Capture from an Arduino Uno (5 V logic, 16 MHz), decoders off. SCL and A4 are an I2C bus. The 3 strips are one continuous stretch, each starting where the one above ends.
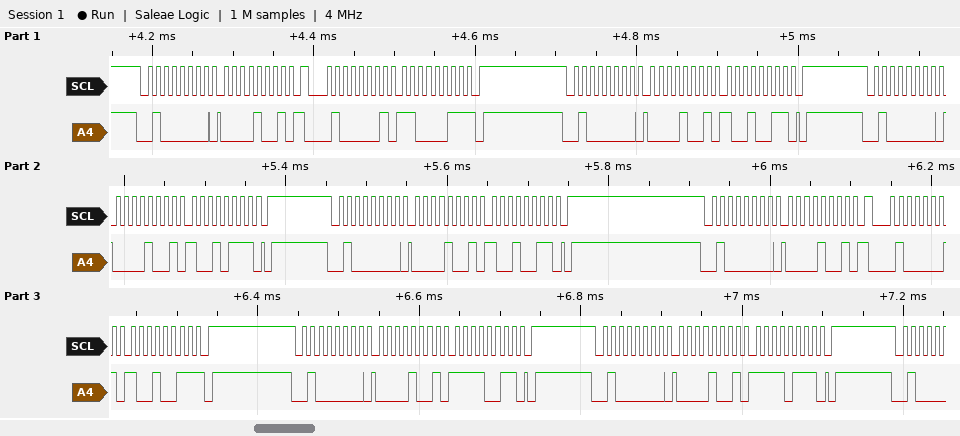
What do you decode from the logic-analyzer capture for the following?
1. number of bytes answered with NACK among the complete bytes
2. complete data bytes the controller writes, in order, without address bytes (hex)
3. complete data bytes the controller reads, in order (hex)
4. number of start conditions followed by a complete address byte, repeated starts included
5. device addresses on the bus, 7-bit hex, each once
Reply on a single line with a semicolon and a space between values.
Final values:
2; 09 09 93 09 97 09 93 09 09 F3 09 F7; C3 93; 9; 0x20
